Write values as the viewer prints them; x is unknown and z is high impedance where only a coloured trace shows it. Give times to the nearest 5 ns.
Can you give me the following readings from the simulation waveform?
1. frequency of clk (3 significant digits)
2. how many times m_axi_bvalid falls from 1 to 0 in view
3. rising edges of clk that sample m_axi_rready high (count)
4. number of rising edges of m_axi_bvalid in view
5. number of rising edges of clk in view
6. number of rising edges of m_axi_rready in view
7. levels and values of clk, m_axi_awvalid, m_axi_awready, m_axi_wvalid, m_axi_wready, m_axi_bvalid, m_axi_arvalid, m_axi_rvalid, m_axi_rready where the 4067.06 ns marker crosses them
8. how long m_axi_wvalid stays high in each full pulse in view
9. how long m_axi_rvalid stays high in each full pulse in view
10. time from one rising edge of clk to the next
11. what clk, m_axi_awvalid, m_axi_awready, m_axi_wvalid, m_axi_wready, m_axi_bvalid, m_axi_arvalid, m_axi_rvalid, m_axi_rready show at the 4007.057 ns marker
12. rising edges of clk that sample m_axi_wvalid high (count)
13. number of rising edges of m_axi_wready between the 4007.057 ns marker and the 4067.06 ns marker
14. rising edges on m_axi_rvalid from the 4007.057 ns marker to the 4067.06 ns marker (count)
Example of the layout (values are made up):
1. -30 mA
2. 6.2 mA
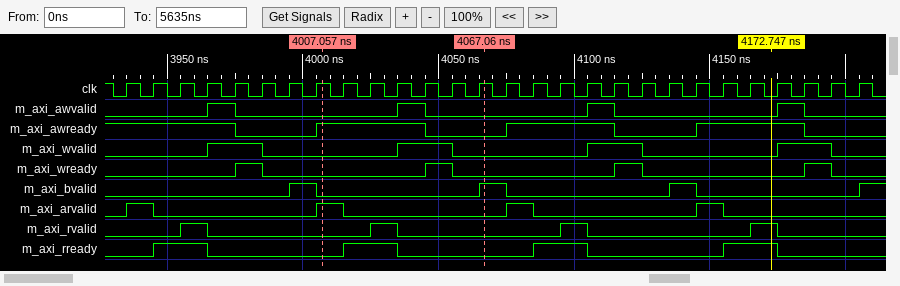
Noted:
1. 100 MHz
2. 3
3. 8
4. 4
5. 28
6. 4
7. clk=1, m_axi_awvalid=0, m_axi_awready=0, m_axi_wvalid=0, m_axi_wready=0, m_axi_bvalid=1, m_axi_arvalid=0, m_axi_rvalid=0, m_axi_rready=0
8. 20 ns, 20 ns, 20 ns, 20 ns
9. 10 ns, 10 ns, 10 ns, 10 ns
10. 10 ns
11. clk=1, m_axi_awvalid=0, m_axi_awready=1, m_axi_wvalid=0, m_axi_wready=0, m_axi_bvalid=0, m_axi_arvalid=1, m_axi_rvalid=0, m_axi_rready=0
12. 8
13. 1
14. 1
